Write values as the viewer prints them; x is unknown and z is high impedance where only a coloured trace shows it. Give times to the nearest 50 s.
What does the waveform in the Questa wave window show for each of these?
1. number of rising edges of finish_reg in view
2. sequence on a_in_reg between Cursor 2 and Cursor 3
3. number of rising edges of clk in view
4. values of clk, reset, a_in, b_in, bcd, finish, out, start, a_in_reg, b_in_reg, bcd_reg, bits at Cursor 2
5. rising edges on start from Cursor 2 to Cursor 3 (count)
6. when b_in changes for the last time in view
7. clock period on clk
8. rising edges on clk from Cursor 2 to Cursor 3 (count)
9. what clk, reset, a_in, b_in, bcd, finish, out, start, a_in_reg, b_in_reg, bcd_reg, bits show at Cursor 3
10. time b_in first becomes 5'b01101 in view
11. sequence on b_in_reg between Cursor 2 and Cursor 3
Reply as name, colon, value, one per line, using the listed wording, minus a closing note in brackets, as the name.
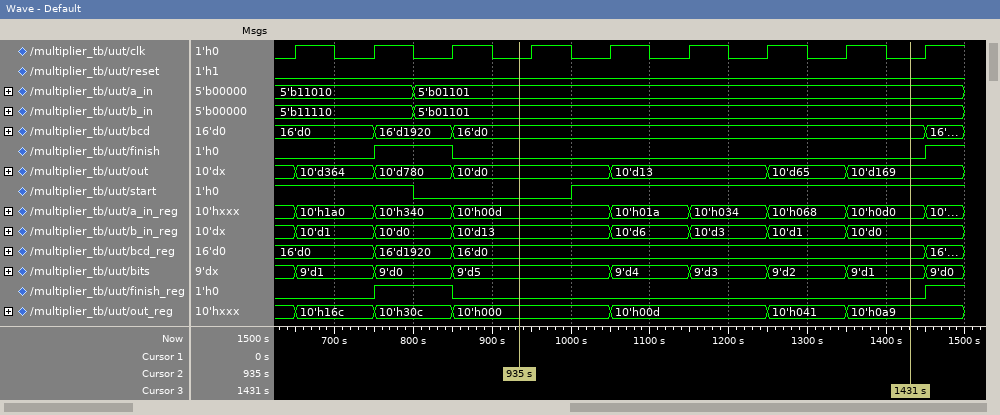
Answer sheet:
number of rising edges of finish_reg in view: 2
sequence on a_in_reg between Cursor 2 and Cursor 3: 10'h00d, 10'h01a, 10'h034, 10'h068, 10'h0d0
number of rising edges of clk in view: 9
values of clk, reset, a_in, b_in, bcd, finish, out, start, a_in_reg, b_in_reg, bcd_reg, bits at Cursor 2: clk=0, reset=0, a_in=5'b01101, b_in=5'b01101, bcd=16'd0, finish=0, out=10'd0, start=0, a_in_reg=10'h00d, b_in_reg=10'd13, bcd_reg=16'd0, bits=9'd5
rising edges on start from Cursor 2 to Cursor 3: 1
when b_in changes for the last time in view: 800 s
clock period on clk: 100 s
rising edges on clk from Cursor 2 to Cursor 3: 5
what clk, reset, a_in, b_in, bcd, finish, out, start, a_in_reg, b_in_reg, bcd_reg, bits show at Cursor 3: clk=0, reset=0, a_in=5'b01101, b_in=5'b01101, bcd=16'd0, finish=0, out=10'd169, start=1, a_in_reg=10'h0d0, b_in_reg=10'd0, bcd_reg=16'd0, bits=9'd1
time b_in first becomes 5'b01101 in view: 800 s
sequence on b_in_reg between Cursor 2 and Cursor 3: 10'd13, 10'd6, 10'd3, 10'd1, 10'd0
